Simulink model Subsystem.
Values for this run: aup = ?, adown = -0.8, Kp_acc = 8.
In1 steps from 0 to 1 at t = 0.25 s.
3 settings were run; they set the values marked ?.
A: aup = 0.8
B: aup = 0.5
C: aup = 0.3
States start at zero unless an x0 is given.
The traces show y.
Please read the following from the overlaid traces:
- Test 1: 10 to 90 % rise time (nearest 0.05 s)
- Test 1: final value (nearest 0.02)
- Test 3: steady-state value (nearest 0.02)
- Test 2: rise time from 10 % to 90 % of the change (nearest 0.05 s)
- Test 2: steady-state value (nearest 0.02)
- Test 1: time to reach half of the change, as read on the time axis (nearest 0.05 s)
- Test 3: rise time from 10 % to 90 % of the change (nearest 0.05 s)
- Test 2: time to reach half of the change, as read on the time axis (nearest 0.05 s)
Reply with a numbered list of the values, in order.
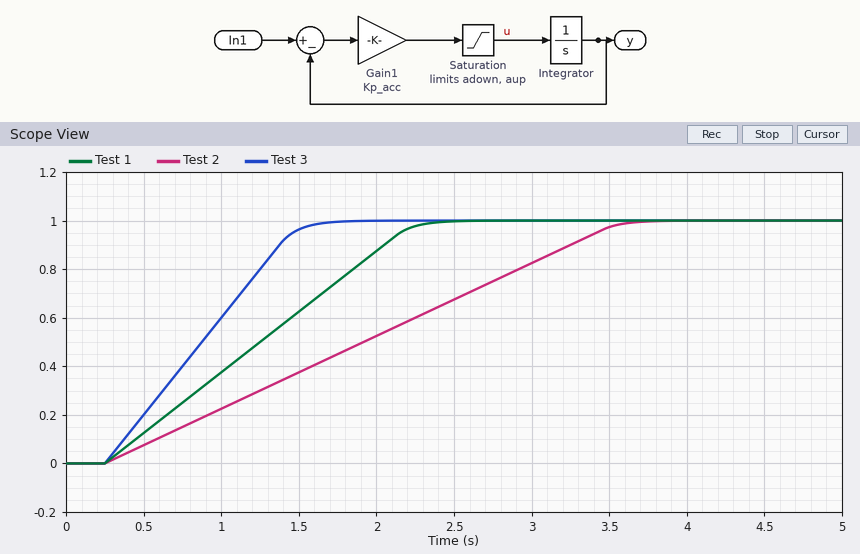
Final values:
1. 1.60 s
2. 1.00
3. 1.00
4. 2.65 s
5. 1.00
6. 1.25 s
7. 1.00 s
8. 1.90 s
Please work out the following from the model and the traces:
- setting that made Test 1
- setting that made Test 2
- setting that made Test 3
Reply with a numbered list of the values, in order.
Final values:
1. B
2. C
3. A
